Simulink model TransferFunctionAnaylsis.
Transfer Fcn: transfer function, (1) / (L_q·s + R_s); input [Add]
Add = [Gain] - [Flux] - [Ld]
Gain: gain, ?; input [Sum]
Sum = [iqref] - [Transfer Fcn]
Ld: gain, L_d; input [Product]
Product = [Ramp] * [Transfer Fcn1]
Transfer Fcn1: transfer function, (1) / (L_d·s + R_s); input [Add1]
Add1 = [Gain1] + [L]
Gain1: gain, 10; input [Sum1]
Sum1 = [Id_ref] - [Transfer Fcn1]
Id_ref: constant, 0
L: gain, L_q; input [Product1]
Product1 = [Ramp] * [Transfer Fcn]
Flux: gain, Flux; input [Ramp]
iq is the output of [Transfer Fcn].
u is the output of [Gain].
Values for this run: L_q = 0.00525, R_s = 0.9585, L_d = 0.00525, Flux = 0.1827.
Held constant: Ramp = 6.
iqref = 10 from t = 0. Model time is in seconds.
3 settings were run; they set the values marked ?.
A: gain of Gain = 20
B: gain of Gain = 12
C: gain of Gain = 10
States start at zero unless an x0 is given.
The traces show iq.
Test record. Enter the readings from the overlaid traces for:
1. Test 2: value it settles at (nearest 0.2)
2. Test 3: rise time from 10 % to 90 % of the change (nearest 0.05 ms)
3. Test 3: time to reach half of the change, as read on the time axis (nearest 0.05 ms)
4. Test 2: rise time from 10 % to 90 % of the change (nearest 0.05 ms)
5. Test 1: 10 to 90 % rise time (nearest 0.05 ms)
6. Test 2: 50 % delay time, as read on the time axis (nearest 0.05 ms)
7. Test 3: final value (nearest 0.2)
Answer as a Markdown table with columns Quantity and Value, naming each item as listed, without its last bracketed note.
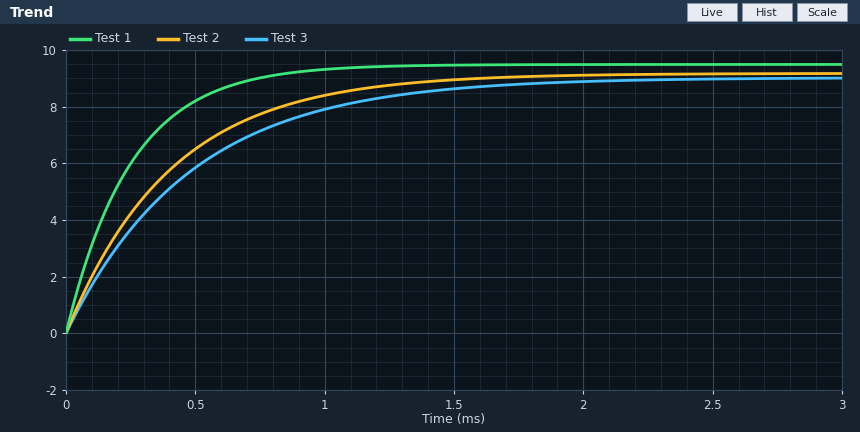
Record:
| Quantity | Value |
|---|---|
| Test 2: value it settles at | 9.2 |
| Test 3: rise time from 10 % to 90 % of the change | 1.05 ms |
| Test 3: time to reach half of the change, as read on the time axis | 0.35 ms |
| Test 2: rise time from 10 % to 90 % of the change | 0.90 ms |
| Test 1: 10 to 90 % rise time | 0.55 ms |
| Test 2: 50 % delay time, as read on the time axis | 0.30 ms |
| Test 3: final value | 9.0 |
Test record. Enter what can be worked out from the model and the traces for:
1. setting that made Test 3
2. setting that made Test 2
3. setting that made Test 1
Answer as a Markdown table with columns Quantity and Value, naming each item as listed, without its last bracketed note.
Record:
| Quantity | Value |
|---|---|
| setting that made Test 3 | C |
| setting that made Test 2 | B |
| setting that made Test 1 | A |
